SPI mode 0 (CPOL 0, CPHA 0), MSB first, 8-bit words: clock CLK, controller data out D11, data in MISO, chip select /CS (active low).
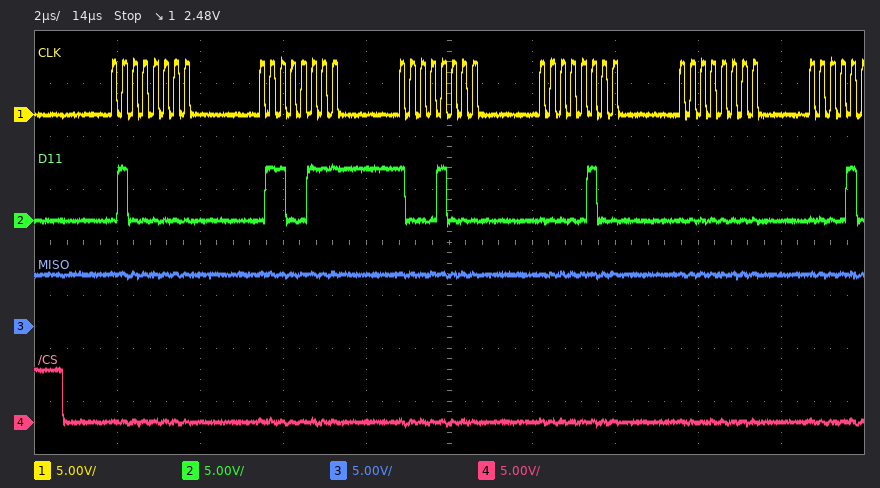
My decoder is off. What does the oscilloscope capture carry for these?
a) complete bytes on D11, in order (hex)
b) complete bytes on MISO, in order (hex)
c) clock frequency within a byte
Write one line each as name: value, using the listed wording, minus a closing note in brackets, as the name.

complete bytes on D11, in order: 40 67 88 04 00
complete bytes on MISO, in order: FF FF FF FF FF
clock frequency within a byte: 4 MHz
